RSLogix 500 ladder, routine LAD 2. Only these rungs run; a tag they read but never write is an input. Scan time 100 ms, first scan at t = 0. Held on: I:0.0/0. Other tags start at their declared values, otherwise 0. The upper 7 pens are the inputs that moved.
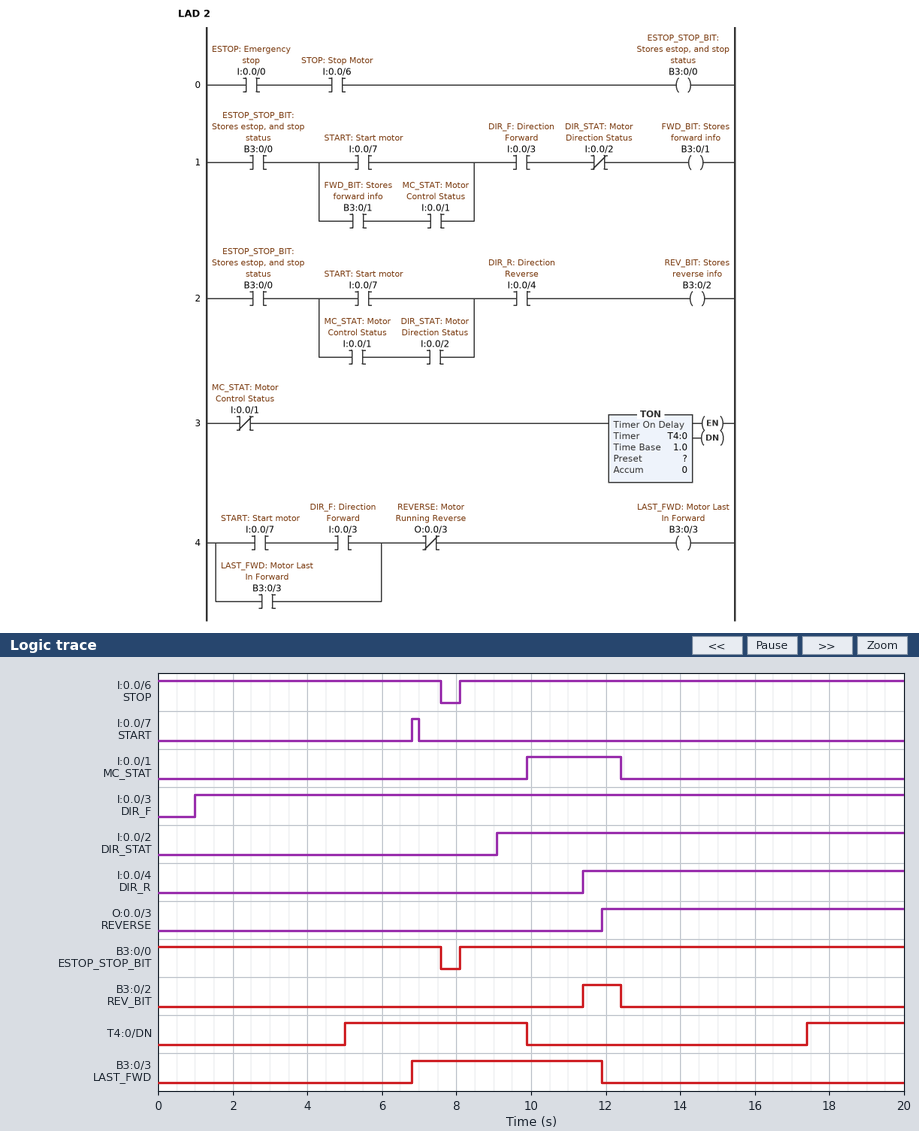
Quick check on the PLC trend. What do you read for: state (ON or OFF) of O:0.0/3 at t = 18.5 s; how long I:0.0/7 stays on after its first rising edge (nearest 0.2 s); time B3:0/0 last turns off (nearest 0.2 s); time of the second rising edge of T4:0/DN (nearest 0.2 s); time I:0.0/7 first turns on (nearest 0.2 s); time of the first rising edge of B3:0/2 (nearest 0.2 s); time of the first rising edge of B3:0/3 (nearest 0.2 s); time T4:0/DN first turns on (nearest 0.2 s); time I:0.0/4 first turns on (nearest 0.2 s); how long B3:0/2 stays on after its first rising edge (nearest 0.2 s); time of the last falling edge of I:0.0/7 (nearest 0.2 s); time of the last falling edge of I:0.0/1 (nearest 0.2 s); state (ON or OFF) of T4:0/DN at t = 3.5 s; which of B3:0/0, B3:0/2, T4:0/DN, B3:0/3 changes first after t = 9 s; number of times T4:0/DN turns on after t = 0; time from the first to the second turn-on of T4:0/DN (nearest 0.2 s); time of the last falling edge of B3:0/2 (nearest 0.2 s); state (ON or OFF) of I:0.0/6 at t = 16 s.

ON
0.2 s
7.6 s
17.4 s
6.8 s
11.4 s
6.8 s
5.0 s
11.4 s
1.0 s
7.0 s
12.4 s
OFF
T4:0/DN
2
12.4 s
12.4 s
ON
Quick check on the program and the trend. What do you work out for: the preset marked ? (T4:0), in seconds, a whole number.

5 s
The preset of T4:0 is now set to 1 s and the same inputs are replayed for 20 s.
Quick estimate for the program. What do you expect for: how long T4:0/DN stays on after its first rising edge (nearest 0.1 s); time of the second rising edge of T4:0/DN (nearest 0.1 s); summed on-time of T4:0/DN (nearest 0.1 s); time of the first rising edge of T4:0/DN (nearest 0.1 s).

8.9 s
13.4 s
15.5 s
1.0 s
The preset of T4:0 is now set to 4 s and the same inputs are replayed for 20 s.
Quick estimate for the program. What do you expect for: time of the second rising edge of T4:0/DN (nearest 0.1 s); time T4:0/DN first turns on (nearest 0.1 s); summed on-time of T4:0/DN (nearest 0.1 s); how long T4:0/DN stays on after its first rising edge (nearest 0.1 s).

16.4 s
4.0 s
9.5 s
5.9 s
